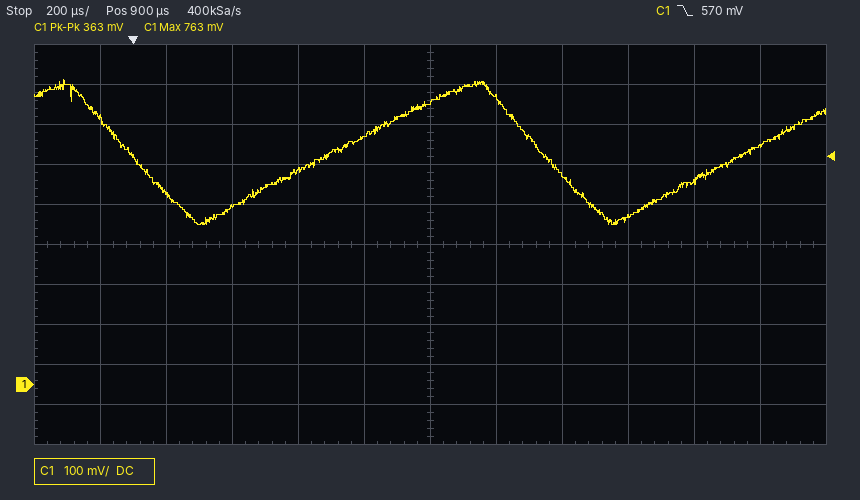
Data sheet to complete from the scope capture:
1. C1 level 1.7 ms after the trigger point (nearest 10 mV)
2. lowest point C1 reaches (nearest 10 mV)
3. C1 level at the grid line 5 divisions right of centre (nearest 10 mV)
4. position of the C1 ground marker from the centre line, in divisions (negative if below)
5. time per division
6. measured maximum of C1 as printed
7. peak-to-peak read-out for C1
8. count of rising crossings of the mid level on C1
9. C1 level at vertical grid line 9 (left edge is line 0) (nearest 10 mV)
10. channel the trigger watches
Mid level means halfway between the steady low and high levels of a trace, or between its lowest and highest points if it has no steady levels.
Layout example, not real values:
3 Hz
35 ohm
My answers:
510 mV
400 mV
600 mV
-3.5 div
200 µs
763 mV
363 mV
2
420 mV
C1
